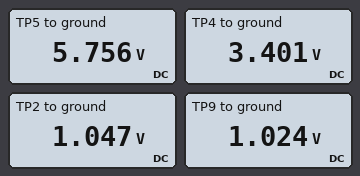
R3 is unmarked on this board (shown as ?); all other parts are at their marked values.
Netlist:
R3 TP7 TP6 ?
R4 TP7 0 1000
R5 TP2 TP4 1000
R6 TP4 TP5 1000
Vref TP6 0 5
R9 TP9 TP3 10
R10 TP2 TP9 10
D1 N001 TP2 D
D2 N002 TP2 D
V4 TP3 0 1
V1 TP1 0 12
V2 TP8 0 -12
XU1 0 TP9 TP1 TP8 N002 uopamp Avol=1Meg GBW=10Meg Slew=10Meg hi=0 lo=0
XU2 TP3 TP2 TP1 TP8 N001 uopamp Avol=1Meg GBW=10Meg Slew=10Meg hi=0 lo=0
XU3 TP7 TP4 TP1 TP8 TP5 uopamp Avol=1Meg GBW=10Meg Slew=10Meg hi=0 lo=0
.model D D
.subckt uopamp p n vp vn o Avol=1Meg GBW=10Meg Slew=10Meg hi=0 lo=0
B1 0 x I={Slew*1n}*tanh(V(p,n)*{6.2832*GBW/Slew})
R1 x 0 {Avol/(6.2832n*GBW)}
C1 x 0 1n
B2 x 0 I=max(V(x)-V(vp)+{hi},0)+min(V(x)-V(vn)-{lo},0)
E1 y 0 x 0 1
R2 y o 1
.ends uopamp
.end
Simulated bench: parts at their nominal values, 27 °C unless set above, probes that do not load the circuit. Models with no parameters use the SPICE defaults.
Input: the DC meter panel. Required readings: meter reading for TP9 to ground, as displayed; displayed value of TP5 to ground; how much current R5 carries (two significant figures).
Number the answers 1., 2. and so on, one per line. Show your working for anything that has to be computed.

1. 1.024 V
2. 5.756 V
3. (3.401 V - 1.047 V) / 1 kΩ = 2.4 mA
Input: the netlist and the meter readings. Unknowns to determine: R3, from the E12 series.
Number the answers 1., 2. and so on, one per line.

1. 470 Ω
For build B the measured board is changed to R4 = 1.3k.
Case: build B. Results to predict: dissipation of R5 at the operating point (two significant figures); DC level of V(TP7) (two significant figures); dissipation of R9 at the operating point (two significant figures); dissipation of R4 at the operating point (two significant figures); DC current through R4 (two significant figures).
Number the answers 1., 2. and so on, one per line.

1. 6.9 mW
2. 3.7 V
3. 69 µW
4. 10 mW
5. 2.8 mA
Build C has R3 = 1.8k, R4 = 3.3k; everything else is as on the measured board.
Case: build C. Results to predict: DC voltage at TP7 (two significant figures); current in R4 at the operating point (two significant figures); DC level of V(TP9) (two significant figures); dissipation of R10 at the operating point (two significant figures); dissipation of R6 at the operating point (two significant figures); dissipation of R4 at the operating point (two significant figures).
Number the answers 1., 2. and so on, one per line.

1. 3.2 V
2. 980 µA
3. 1.0 V
4. 48 µW
5. 4.8 mW
6. 3.2 mW
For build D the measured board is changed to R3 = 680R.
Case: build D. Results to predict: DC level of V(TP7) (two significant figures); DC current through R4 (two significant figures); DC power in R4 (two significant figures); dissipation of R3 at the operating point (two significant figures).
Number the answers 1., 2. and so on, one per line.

1. 3.0 V
2. 3.0 mA
3. 8.9 mW
4. 6.0 mW
